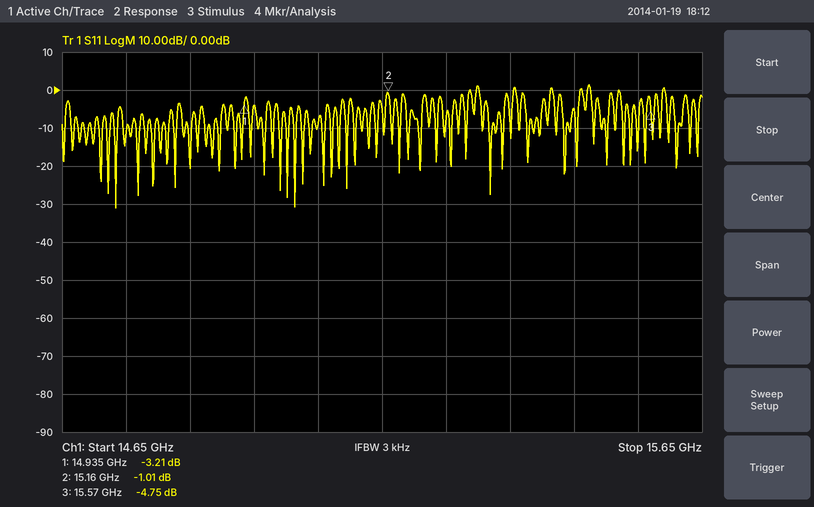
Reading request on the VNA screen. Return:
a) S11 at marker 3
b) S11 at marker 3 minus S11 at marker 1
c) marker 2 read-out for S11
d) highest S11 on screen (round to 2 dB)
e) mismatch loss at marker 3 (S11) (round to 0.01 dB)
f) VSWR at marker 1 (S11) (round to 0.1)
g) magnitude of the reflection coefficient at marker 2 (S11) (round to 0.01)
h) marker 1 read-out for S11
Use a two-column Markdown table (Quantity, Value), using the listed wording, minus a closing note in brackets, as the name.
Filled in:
| Quantity | Value |
|---|---|
| S11 at marker 3 | -4.75 dB |
| S11 at marker 3 minus S11 at marker 1 | -1.54 dB |
| marker 2 read-out for S11 | -1.01 dB |
| highest S11 on screen | 2 dB |
| mismatch loss at marker 3 (S11) | 1.77 dB |
| VSWR at marker 1 (S11) | 5.5 |
| magnitude of the reflection coefficient at marker 2 (S11) | 0.89 |
| marker 1 read-out for S11 | -3.21 dB |
